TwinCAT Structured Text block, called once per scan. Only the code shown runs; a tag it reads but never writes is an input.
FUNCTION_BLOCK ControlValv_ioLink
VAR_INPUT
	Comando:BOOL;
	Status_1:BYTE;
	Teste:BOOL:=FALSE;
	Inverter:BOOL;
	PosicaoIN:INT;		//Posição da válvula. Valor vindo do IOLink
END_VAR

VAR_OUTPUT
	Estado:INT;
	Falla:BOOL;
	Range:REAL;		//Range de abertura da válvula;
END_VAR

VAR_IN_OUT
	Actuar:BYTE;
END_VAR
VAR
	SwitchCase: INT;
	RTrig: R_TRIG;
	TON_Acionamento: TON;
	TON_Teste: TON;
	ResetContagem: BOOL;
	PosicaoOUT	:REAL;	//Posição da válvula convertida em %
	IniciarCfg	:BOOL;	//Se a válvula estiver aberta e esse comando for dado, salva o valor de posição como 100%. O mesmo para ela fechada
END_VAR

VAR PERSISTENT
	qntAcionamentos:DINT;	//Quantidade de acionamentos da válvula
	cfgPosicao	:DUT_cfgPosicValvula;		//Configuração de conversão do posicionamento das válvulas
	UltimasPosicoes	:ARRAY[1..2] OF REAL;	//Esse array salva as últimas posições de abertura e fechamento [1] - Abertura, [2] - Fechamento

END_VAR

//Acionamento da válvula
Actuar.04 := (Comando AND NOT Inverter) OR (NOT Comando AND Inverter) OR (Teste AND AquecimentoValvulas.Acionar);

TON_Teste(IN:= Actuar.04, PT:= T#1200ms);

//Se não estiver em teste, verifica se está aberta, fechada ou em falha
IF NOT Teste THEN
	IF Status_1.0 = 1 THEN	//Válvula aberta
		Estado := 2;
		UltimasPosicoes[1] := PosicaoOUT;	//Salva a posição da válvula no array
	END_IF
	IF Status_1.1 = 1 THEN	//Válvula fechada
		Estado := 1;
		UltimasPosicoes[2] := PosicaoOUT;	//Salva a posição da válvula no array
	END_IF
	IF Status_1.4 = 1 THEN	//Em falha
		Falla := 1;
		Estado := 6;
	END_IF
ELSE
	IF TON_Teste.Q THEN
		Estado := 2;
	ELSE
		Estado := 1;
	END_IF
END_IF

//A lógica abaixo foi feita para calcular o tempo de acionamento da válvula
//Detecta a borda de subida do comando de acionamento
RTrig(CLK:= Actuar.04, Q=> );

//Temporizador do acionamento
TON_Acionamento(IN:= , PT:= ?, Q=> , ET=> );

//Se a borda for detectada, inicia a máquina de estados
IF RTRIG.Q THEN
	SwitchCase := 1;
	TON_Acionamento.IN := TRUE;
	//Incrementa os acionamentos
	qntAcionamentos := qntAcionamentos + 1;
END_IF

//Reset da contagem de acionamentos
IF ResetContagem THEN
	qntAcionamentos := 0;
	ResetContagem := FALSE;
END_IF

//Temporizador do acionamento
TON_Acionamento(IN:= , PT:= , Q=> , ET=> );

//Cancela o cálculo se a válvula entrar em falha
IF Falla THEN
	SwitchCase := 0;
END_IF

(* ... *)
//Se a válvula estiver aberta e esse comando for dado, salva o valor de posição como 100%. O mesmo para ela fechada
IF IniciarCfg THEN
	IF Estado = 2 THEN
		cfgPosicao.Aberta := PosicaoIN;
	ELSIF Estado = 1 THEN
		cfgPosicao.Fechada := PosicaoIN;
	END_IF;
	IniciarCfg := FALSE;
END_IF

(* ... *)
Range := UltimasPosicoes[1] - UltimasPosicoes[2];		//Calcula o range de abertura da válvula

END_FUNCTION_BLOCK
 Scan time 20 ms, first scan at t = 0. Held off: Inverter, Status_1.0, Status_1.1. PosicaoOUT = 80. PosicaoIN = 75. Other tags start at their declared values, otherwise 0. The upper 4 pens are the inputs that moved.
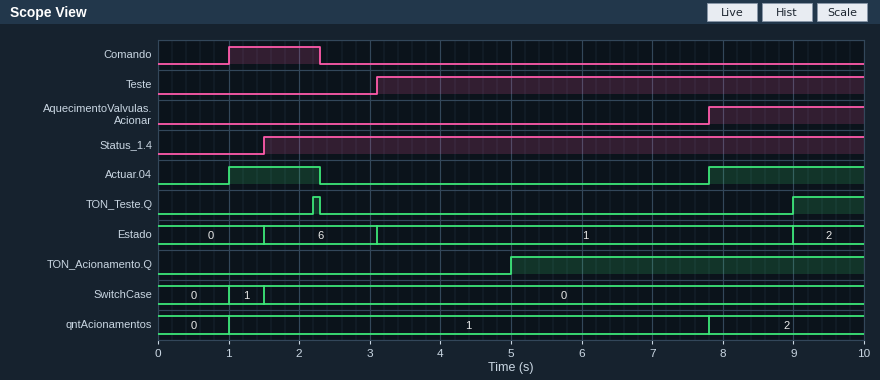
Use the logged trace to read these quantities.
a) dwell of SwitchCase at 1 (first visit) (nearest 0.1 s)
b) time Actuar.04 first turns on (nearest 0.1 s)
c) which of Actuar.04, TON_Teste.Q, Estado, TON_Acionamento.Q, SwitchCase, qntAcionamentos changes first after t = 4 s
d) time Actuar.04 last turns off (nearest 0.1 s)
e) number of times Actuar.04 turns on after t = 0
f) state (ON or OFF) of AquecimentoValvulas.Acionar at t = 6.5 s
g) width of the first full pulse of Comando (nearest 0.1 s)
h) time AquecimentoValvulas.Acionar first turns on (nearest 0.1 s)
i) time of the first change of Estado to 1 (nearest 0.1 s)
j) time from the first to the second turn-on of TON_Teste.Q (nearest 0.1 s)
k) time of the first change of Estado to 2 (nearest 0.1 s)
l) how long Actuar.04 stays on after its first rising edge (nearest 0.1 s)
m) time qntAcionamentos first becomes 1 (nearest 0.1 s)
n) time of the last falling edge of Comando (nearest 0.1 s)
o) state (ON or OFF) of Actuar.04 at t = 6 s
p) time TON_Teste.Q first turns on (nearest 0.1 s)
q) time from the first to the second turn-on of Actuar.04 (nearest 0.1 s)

0.5 s
1.0 s
TON_Acionamento.Q
2.3 s
2
OFF
1.3 s
7.8 s
3.1 s
6.8 s
9.0 s
1.3 s
1.0 s
2.3 s
OFF
2.2 s
6.8 s
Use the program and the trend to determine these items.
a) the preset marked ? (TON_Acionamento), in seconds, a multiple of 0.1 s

4.0 s
